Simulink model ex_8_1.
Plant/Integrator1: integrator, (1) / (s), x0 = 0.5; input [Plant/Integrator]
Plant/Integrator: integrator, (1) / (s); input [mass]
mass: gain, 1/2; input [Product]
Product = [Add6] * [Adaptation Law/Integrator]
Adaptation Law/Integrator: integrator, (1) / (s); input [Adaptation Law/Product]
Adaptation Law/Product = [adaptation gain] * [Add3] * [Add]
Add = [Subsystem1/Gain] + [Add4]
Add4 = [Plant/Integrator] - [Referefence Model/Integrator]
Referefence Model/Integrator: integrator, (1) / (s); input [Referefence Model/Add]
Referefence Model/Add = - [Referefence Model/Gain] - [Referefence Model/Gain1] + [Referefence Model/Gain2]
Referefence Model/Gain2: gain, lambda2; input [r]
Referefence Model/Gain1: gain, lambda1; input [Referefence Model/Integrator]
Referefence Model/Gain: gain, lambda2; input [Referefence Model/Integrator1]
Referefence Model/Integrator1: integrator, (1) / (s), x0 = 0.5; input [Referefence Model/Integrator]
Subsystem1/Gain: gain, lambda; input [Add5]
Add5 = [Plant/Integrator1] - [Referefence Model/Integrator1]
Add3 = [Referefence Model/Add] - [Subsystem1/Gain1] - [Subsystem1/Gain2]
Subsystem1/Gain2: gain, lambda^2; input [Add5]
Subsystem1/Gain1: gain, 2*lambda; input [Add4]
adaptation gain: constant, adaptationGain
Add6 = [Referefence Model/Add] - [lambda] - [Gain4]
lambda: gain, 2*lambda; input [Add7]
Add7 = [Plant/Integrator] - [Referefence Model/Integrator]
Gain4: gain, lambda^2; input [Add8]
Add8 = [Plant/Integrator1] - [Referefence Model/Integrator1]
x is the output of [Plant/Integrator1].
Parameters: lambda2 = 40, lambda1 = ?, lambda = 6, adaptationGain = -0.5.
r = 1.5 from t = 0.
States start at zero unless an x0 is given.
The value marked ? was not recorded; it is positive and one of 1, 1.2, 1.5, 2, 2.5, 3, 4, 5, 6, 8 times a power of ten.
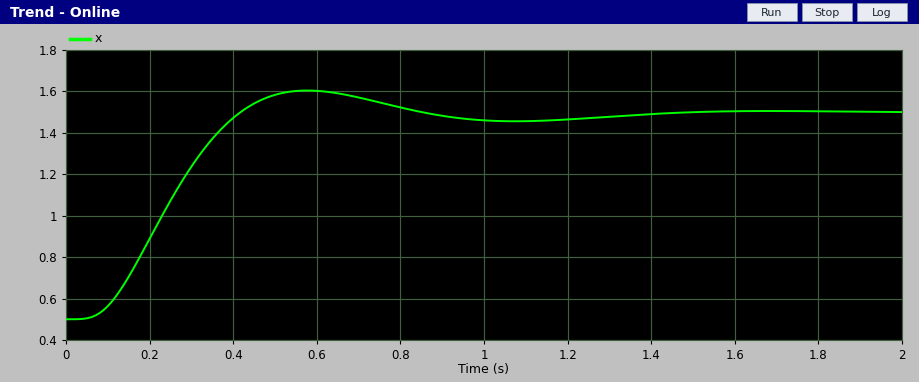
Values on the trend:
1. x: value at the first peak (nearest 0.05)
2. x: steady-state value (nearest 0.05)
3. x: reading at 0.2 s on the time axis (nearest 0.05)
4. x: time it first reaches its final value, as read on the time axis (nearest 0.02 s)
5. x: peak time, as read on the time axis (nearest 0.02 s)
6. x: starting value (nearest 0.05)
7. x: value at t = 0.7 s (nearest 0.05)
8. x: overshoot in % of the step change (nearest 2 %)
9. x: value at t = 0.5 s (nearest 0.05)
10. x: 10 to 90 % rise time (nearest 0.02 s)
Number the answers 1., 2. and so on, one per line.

1. 1.60
2. 1.50
3. 0.90
4. 0.42 s
5. 0.58 s
6. 0.50
7. 1.55
8. 10 %
9. 1.60
10. 0.24 s
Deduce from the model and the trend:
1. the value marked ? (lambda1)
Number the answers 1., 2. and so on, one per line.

1. 6
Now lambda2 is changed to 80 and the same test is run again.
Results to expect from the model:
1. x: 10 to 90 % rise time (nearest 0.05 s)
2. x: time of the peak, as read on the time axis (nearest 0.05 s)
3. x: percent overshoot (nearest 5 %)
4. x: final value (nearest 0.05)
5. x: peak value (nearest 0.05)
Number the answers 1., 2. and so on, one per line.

1. 0.15 s
2. 0.35 s
3. 20 %
4. 1.50
5. 1.70
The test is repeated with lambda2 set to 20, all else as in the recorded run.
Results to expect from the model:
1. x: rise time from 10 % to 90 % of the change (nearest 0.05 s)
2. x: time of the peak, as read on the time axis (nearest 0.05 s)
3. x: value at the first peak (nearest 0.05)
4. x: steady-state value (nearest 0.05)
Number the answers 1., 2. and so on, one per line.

1. 0.45 s
2. 1.00 s
3. 1.55
4. 1.50
